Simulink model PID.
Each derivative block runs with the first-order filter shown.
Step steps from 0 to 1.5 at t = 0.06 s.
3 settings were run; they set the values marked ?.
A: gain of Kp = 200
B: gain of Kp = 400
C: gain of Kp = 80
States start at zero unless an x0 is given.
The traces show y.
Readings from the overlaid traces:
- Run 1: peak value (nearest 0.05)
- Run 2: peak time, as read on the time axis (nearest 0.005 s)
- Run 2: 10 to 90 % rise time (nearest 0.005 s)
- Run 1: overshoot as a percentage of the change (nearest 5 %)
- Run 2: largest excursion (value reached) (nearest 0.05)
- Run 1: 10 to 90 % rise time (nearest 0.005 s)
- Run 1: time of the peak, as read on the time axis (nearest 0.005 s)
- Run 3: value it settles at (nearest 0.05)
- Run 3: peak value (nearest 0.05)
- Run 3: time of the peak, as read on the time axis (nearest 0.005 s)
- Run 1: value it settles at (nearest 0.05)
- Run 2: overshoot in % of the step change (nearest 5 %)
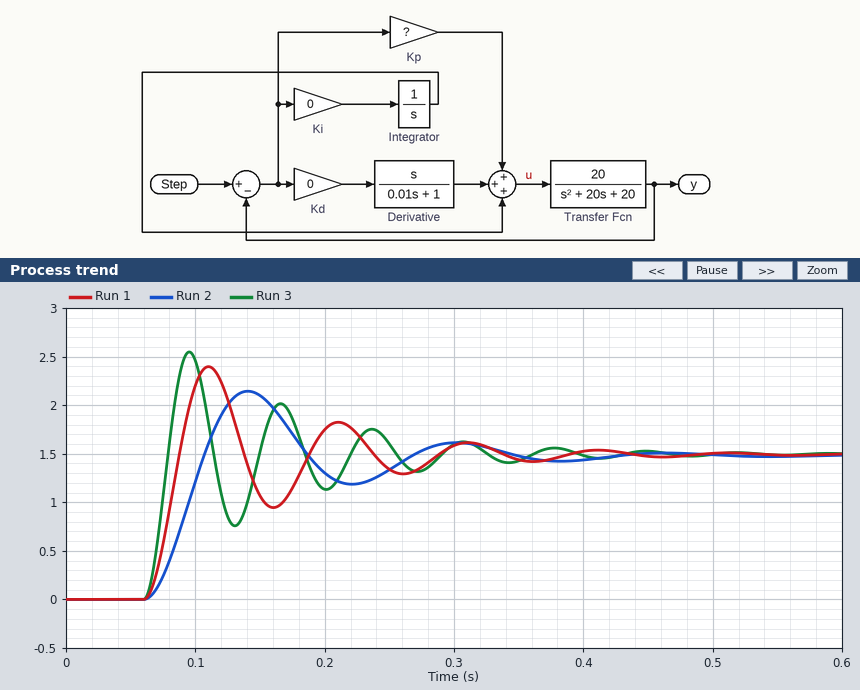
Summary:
2.40
0.140 s
0.030 s
60 %
2.15
0.020 s
0.110 s
1.50
2.55
0.095 s
1.50
45 %
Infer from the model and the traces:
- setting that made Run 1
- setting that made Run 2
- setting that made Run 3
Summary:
A
C
B
